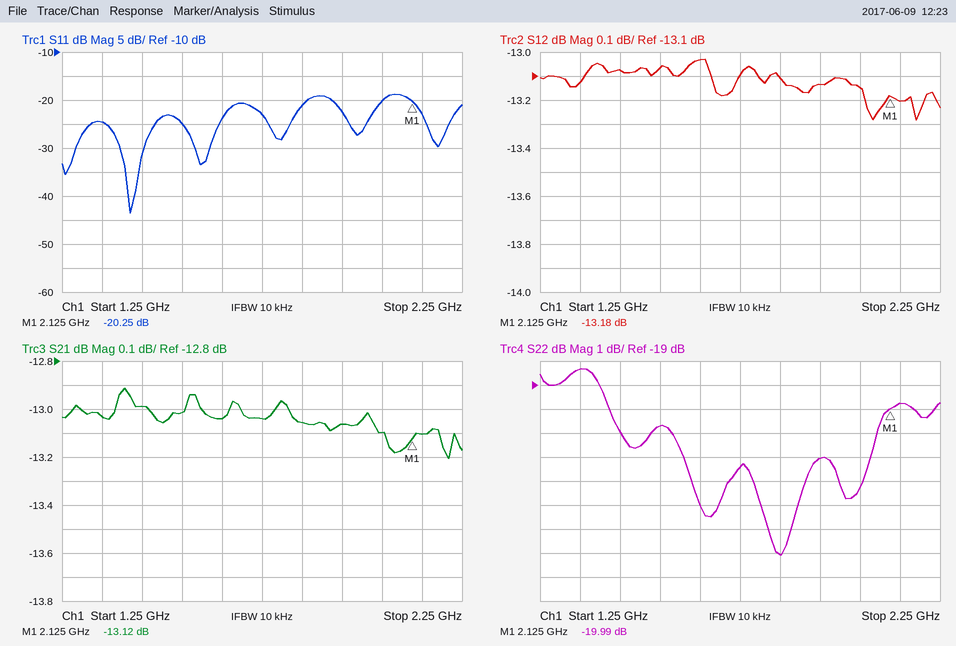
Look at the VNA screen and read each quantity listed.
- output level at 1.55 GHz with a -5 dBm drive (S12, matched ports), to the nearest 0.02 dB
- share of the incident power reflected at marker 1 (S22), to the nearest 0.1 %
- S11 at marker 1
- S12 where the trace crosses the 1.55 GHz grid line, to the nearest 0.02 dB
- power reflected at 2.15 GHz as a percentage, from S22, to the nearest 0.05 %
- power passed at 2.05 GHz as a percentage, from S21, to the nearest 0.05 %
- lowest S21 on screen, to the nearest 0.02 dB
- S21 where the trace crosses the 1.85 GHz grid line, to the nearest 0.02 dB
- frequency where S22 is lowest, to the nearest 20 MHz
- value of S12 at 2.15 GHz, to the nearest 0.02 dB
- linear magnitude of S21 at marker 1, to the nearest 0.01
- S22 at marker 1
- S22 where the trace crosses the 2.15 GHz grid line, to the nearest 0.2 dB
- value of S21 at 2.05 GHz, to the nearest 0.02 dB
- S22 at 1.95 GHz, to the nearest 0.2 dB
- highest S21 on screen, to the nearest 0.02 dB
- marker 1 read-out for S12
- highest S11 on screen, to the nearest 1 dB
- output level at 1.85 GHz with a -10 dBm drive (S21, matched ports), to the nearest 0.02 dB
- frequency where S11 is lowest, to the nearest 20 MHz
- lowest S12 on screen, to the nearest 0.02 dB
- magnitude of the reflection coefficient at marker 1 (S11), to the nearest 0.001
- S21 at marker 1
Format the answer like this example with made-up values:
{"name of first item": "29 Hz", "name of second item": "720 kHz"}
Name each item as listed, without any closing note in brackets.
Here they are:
{"output level at 1.55 GHz with a -5 dBm drive (S12, matched ports), to the nearest 0.02 dB": "-18.06 dBm", "share of the incident power reflected at marker 1 (S22), to the nearest 0.1 %": "1.0 %", "S11 at marker 1": "-20.25 dB", "S12 where the trace crosses the 1.55 GHz grid line, to the nearest 0.02 dB": "-13.06 dB", "power reflected at 2.15 GHz as a percentage, from S22, to the nearest 0.05 %": "1.05 %", "power passed at 2.05 GHz as a percentage, from S21, to the nearest 0.05 %": "4.90 %", "lowest S21 on screen, to the nearest 0.02 dB": "-13.20 dB", "S21 where the trace crosses the 1.85 GHz grid line, to the nearest 0.02 dB": "-13.06 dB", "frequency where S22 is lowest, to the nearest 20 MHz": "1.86 GHz", "value of S12 at 2.15 GHz, to the nearest 0.02 dB": "-13.20 dB", "linear magnitude of S21 at marker 1, to the nearest 0.01": "0.22", "S22 at marker 1": "-19.99 dB", "S22 where the trace crosses the 2.15 GHz grid line, to the nearest 0.2 dB": "-19.8 dB", "value of S21 at 2.05 GHz, to the nearest 0.02 dB": "-13.10 dB", "S22 at 1.95 GHz, to the nearest 0.2 dB": "-22.0 dB", "highest S21 on screen, to the nearest 0.02 dB": "-12.92 dB", "marker 1 read-out for S12": "-13.18 dB", "highest S11 on screen, to the nearest 1 dB": "-19 dB", "output level at 1.85 GHz with a -10 dBm drive (S21, matched ports), to the nearest 0.02 dB": "-23.06 dBm", "frequency where S11 is lowest, to the nearest 20 MHz": "1.42 GHz", "lowest S12 on screen, to the nearest 0.02 dB": "-13.28 dB", "magnitude of the reflection coefficient at marker 1 (S11), to the nearest 0.001": "0.097", "S21 at marker 1": "-13.12 dB"}
